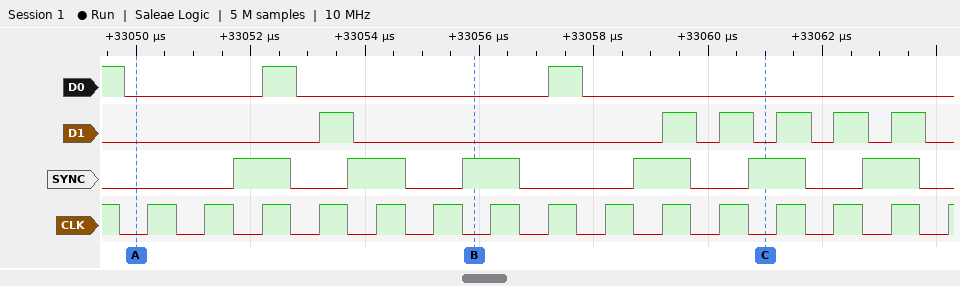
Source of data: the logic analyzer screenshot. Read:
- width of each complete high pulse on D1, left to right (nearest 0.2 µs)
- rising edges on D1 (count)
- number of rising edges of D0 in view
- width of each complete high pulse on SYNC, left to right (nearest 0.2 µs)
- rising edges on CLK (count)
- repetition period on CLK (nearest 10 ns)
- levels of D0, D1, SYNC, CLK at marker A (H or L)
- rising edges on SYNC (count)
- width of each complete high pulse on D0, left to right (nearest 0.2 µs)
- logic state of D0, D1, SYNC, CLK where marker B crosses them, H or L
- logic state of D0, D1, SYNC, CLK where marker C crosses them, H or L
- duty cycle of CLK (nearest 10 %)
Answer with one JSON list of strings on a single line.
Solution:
["0.6 µs, 0.6 µs, 0.6 µs, 0.6 µs, 0.6 µs, 0.6 µs", "6", "2", "1 µs, 1 µs, 1 µs, 1 µs, 1 µs, 1 µs", "15", "1000 ns", "D0=L, D1=L, SYNC=L, CLK=L", "6", "0.6 µs, 0.6 µs", "D0=L, D1=L, SYNC=H, CLK=L", "D0=L, D1=L, SYNC=H, CLK=L", "50 %"]
